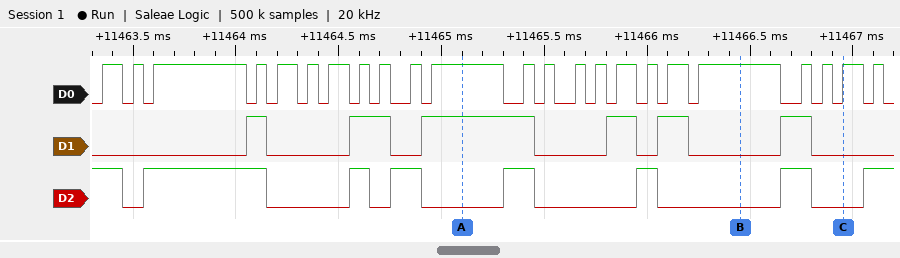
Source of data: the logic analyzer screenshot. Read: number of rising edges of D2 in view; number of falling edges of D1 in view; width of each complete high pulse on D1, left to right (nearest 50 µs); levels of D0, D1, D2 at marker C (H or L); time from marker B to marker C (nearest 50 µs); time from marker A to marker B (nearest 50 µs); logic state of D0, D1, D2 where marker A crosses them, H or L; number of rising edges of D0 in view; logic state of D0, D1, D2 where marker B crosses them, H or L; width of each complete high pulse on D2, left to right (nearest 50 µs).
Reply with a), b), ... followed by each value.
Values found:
a) 7
b) 6
c) 100 µs, 200 µs, 550 µs, 150 µs, 150 µs, 150 µs
d) D0=H, D1=L, D2=L
e) 500 µs
f) 1350 µs
g) D0=H, D1=H, D2=L
h) 23
i) D0=H, D1=L, D2=L
j) 600 µs, 100 µs, 150 µs, 150 µs, 100 µs, 150 µs
